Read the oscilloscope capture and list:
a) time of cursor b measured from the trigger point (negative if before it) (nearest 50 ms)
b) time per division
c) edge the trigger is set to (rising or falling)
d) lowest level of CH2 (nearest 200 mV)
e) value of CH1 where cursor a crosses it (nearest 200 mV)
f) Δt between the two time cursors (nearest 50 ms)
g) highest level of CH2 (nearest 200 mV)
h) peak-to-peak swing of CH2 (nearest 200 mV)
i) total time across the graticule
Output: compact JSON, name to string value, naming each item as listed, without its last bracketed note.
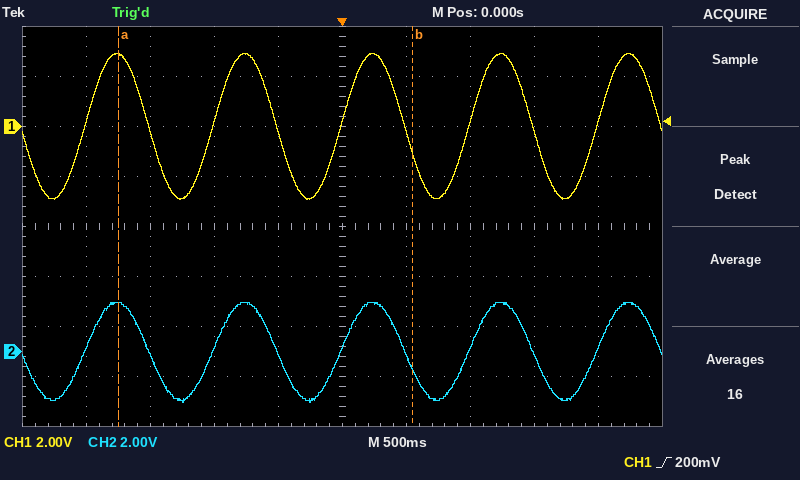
{"time of cursor b measured from the trigger point (negative if before it)": "+550 ms", "time per division": "500 ms", "edge the trigger is set to": "rising", "lowest level of CH2": "-2.0 V", "value of CH1 where cursor a crosses it": "2.8 V", "Δt between the two time cursors": "2.30 s", "highest level of CH2": "2.0 V", "peak-to-peak swing of CH2": "4.0 V", "total time across the graticule": "5 s"}
